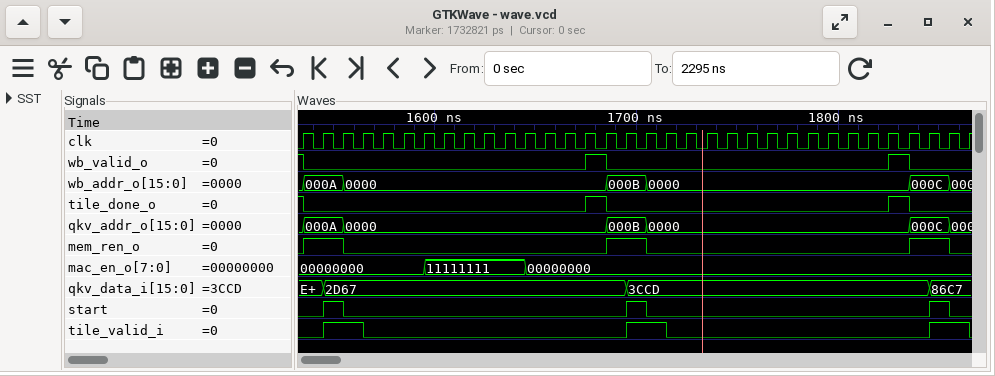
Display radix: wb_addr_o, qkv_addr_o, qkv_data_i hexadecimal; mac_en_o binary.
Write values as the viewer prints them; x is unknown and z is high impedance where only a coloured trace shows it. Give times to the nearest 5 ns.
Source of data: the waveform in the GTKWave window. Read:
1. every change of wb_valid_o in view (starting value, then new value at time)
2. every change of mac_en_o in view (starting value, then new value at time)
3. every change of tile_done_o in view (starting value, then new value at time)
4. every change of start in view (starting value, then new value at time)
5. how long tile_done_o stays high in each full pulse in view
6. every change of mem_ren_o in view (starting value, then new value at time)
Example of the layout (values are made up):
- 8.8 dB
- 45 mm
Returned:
- 1, 0 at 1535 ns, 1 at 1675 ns, 0 at 1685 ns, 1 at 1825 ns, 0 at 1835 ns
- 00000000, 11111111 at 1595 ns, 00000000 at 1645 ns
- 1, 0 at 1535 ns, 1 at 1675 ns, 0 at 1685 ns, 1 at 1825 ns, 0 at 1835 ns
- 0, 1 at 1545 ns, 0 at 1555 ns, 1 at 1695 ns, 0 at 1705 ns, 1 at 1845 ns, 0 at 1855 ns
- 10 ns, 10 ns
- 0, 1 at 1535 ns, 0 at 1555 ns, 1 at 1685 ns, 0 at 1705 ns, 1 at 1835 ns, 0 at 1855 ns
